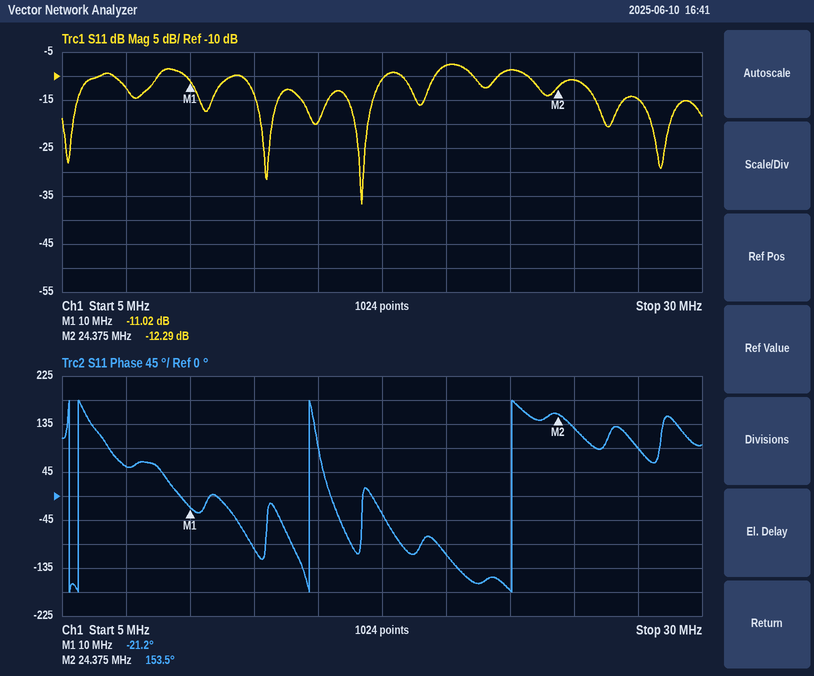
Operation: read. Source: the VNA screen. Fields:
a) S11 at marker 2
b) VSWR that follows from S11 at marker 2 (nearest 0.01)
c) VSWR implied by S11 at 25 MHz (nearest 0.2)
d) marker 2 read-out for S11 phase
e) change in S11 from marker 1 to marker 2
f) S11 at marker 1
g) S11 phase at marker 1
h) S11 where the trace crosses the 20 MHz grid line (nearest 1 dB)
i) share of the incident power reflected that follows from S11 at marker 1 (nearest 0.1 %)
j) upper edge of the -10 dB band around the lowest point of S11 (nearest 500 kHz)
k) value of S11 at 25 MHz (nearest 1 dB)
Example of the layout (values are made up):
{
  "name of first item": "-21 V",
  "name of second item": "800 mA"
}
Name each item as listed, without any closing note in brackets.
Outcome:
{
  "S11 at marker 2": "-12.29 dB",
  "VSWR that follows from S11 at marker 2": "1.64",
  "VSWR implied by S11 at 25 MHz": "1.8",
  "marker 2 read-out for S11 phase": "153.5°",
  "change in S11 from marker 1 to marker 2": "-1.27 dB",
  "S11 at marker 1": "-11.02 dB",
  "S11 phase at marker 1": "-21.2°",
  "S11 where the trace crosses the 20 MHz grid line": "-8 dB",
  "share of the incident power reflected that follows from S11 at marker 1": "7.9 %",
  "upper edge of the -10 dB band around the lowest point of S11": "17.5 MHz",
  "value of S11 at 25 MHz": "-11 dB"
}
